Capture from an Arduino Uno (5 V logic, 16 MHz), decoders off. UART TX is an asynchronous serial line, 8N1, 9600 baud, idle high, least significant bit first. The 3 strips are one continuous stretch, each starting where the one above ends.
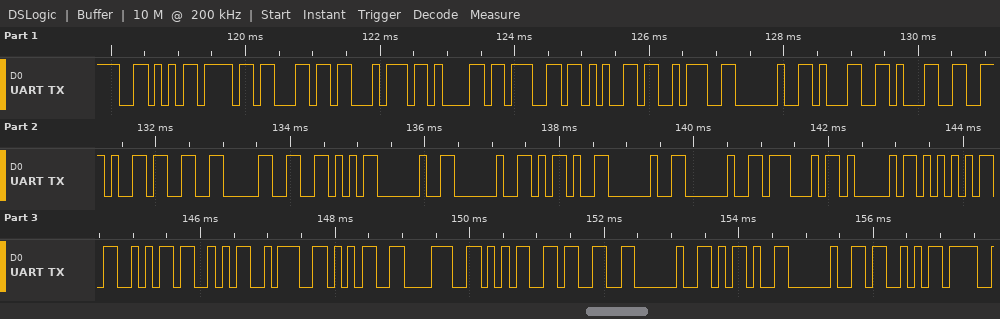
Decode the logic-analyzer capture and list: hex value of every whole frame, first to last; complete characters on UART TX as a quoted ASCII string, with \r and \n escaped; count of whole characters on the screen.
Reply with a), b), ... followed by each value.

a) 56 6F 6C 74 61 67 65 3A 20 31 31 2E 33 30 56 20 20 2D 20 20 47 41 55 53 53 3A 35 38 35 33 20 2D 20 53
b) "Voltage: 11.30V  -  GAUSS:5853 - S"
c) 34
